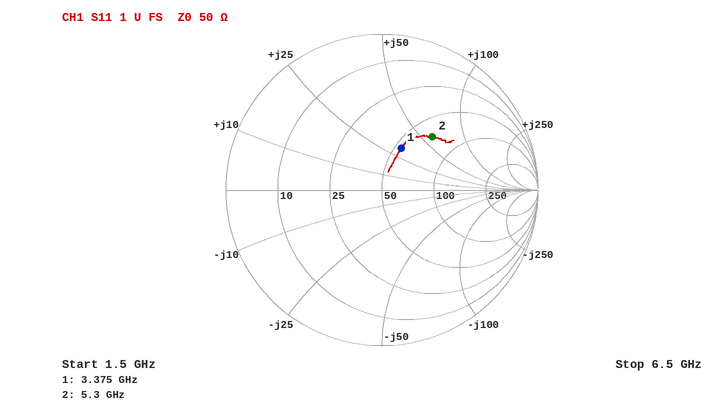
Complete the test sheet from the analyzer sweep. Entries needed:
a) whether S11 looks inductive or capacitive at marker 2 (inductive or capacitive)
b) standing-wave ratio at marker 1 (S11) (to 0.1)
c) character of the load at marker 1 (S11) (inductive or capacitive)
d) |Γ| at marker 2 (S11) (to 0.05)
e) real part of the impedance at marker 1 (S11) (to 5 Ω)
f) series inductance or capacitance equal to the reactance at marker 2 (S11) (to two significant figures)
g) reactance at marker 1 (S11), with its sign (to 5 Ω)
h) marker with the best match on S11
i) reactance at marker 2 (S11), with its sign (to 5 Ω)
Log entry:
inductive
1.8
inductive
0.45
55 Ω
1.8 nH
+30 Ω
marker 1
+60 Ω
